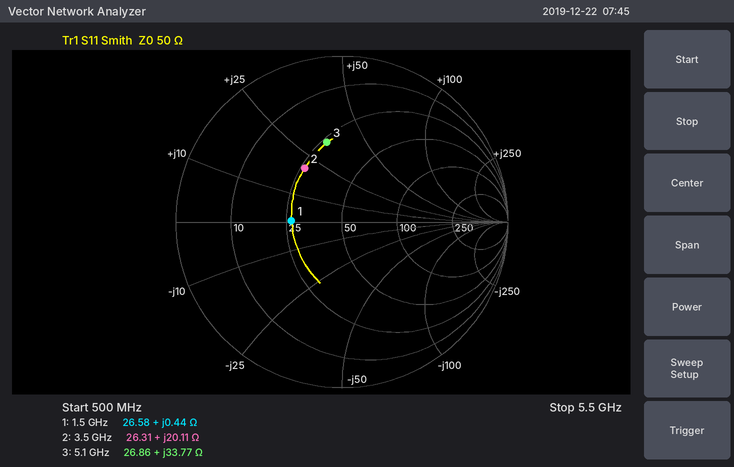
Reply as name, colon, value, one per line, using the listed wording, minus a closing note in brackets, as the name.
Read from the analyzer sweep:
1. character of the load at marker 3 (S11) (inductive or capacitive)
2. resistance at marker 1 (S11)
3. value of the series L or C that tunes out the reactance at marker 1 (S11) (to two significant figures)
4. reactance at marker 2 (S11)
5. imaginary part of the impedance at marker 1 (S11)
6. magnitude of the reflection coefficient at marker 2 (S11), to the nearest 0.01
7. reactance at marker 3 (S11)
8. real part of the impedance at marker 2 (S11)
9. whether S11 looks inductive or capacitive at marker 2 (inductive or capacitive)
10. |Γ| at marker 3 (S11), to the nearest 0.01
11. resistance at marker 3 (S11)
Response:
character of the load at marker 3 (S11): inductive
resistance at marker 1: 26.58 Ω
value of the series L or C that tunes out the reactance at marker 1 (S11): 240 pF
reactance at marker 2: +20.11 Ω
imaginary part of the impedance at marker 1: +0.44 Ω
magnitude of the reflection coefficient at marker 2 (S11), to the nearest 0.01: 0.39
reactance at marker 3: +33.77 Ω
real part of the impedance at marker 2: 26.31 Ω
whether S11 looks inductive or capacitive at marker 2: inductive
|Γ| at marker 3 (S11), to the nearest 0.01: 0.49
resistance at marker 3: 26.86 Ω
